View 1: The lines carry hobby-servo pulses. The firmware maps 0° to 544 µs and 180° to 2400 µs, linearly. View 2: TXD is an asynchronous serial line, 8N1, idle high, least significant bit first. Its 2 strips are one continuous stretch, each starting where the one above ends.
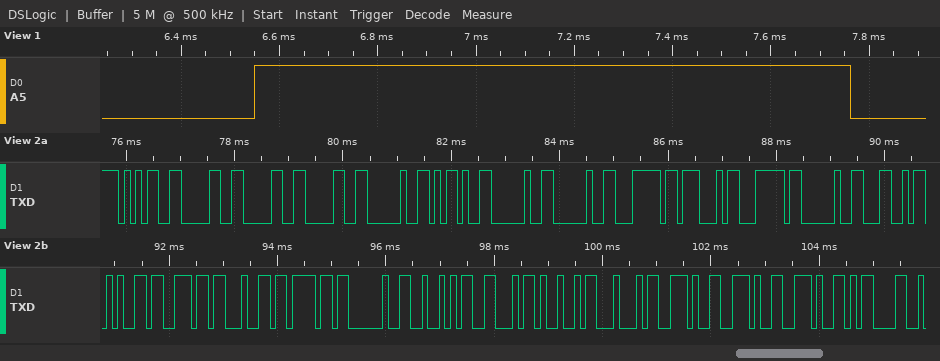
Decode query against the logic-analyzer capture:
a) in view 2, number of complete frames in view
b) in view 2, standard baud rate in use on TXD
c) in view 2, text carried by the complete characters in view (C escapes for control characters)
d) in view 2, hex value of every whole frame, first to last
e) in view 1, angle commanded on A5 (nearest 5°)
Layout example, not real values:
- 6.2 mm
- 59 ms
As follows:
- 26
- 9600 baud
- "5000 -  |G| Lendo RFID...\r"
- 35 30 30 30 20 2D 20 20 7C 47 7C 20 4C 65 6E 64 6F 20 52 46 49 44 2E 2E 2E 0D
- 65°
